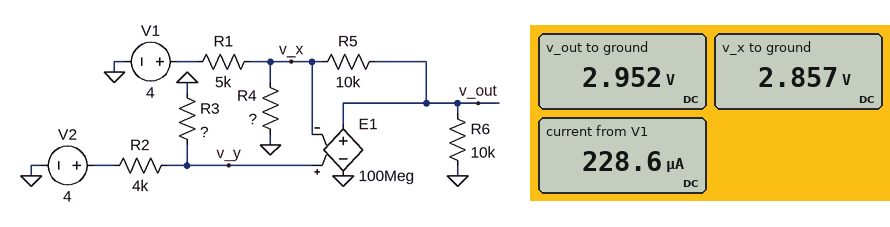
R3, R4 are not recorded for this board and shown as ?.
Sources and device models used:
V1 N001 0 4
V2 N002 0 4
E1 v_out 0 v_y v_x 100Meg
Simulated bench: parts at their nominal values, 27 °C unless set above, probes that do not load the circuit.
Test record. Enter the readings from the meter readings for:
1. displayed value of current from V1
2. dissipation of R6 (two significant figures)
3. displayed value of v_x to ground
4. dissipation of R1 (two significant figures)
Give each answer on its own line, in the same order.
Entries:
228.6 µA
870 µW
2.857 V
260 µW
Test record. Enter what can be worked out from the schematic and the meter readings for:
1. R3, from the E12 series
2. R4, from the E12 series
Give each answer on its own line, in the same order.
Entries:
10 kΩ
12 kΩ
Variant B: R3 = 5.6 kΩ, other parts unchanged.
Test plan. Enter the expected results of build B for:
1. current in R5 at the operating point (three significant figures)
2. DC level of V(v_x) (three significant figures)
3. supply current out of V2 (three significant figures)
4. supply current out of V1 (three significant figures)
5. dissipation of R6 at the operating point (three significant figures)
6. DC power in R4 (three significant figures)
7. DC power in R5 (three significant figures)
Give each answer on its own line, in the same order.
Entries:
139 µA
2.33 V
417 µA
333 µA
89.2 µW
454 µW
193 µW
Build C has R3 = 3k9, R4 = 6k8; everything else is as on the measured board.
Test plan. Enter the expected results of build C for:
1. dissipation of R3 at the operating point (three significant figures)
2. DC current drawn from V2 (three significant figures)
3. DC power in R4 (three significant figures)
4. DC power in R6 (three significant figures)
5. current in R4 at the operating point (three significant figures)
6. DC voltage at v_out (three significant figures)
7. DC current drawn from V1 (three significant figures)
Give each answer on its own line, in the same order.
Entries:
1.00 mW
506 µA
573 µW
68.6 µW
290 µA
828 mV
405 µA
